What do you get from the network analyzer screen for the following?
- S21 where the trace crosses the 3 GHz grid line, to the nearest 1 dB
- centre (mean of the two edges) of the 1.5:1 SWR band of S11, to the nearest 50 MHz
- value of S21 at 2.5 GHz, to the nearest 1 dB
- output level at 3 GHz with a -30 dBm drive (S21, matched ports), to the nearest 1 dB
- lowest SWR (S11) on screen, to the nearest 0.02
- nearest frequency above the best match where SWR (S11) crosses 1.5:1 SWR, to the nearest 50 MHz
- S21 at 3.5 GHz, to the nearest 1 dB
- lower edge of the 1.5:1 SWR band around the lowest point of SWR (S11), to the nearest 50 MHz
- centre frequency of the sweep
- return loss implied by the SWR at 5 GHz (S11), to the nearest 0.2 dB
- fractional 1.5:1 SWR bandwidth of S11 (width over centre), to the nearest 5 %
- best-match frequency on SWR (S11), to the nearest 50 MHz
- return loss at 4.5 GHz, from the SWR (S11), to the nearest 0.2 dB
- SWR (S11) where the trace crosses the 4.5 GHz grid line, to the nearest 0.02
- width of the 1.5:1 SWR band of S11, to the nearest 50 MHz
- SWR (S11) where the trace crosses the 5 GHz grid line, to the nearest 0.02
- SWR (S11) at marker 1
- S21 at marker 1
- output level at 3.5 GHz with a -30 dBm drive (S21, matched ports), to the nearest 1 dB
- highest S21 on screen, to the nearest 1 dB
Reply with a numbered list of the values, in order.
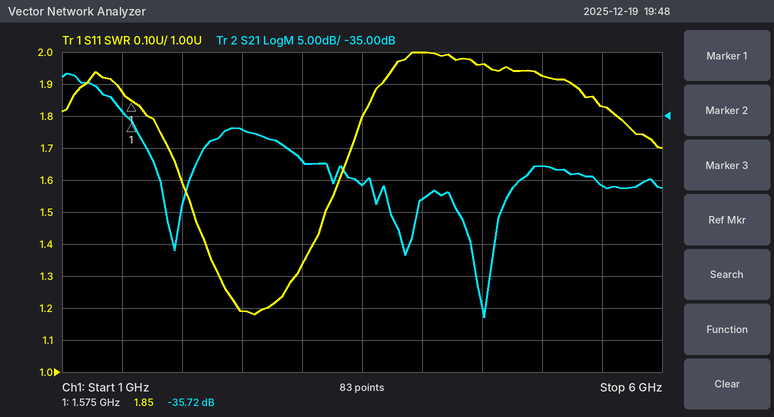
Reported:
1. -42 dB
2. 2.65 GHz
3. -37 dB
4. -72 dBm
5. 1.18
6. 3.20 GHz
7. -46 dB
8. 2.10 GHz
9. 3.5 GHz
10. 10.0 dB
11. 40 %
12. 2.60 GHz
13. 9.8 dB
14. 1.96
15. 1.10 GHz
16. 1.92
17. 1.85
18. -35.72 dB
19. -76 dBm
20. -28 dB
